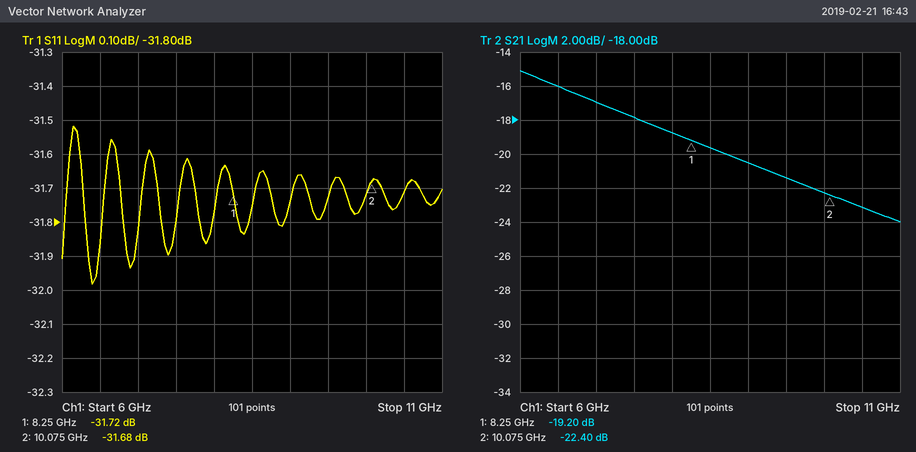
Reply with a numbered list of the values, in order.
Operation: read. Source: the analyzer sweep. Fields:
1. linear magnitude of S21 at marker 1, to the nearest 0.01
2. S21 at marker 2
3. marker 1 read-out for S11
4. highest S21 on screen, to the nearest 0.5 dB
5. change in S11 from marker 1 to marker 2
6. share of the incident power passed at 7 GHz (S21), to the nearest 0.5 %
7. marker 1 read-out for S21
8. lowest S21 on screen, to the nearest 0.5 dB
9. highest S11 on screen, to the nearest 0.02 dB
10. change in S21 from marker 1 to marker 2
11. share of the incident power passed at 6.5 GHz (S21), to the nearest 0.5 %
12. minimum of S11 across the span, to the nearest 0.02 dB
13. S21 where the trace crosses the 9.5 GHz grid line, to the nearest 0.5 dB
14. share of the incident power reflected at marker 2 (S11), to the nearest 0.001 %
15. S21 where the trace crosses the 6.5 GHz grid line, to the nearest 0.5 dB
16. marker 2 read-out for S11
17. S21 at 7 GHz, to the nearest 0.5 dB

1. 0.11
2. -22.40 dB
3. -31.72 dB
4. -15.0 dB
5. 0.04 dB
6. 2.0 %
7. -19.20 dB
8. -24.0 dB
9. -31.52 dB
10. -3.20 dB
11. 2.5 %
12. -31.98 dB
13. -21.5 dB
14. 0.068 %
15. -16.0 dB
16. -31.68 dB
17. -17.0 dB
